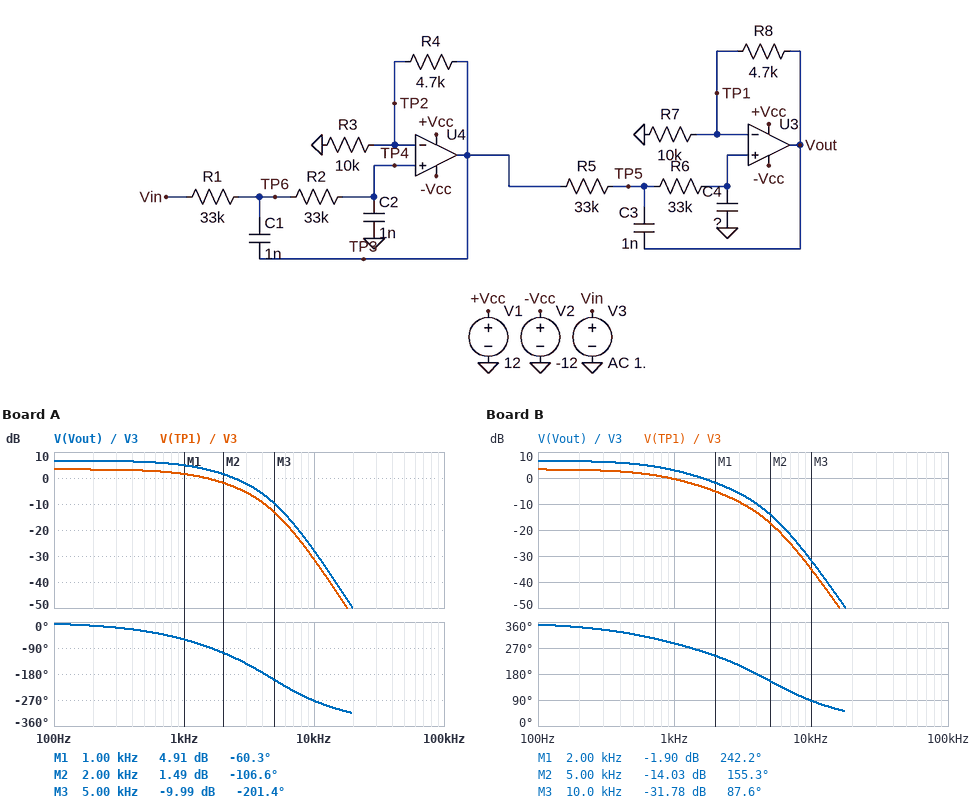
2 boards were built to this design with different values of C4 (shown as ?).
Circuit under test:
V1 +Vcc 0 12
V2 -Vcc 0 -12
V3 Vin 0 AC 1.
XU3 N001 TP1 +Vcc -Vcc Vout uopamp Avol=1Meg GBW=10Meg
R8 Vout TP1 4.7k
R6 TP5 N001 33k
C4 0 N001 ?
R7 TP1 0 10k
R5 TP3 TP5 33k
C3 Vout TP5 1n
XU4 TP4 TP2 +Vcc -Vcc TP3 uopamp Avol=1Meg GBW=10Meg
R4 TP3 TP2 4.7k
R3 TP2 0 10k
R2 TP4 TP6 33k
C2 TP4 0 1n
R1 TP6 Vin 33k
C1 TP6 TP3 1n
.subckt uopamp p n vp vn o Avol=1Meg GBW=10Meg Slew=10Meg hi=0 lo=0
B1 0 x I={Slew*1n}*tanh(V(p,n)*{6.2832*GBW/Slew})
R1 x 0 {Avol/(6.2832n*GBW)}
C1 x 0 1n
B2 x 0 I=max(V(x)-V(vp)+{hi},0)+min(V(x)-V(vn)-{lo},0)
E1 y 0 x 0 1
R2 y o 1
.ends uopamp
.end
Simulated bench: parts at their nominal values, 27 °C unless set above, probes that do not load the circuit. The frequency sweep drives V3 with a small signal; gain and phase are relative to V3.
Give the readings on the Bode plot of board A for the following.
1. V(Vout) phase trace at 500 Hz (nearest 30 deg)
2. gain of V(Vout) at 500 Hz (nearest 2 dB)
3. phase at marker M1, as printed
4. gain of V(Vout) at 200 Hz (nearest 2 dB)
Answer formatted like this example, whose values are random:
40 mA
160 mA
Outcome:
-30 deg
6 dB
-60.3 deg
6 dB
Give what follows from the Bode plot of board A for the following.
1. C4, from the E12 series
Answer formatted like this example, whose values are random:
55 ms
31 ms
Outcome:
2.2 nF
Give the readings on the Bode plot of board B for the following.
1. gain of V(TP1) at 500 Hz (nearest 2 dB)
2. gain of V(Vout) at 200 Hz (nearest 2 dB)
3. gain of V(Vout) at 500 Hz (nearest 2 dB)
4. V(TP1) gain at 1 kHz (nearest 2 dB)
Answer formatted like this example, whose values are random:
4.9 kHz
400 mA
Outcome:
2 dB
6 dB
6 dB
0 dB
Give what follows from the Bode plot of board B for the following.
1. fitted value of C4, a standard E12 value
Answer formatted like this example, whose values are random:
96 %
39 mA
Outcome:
3.3 nF
